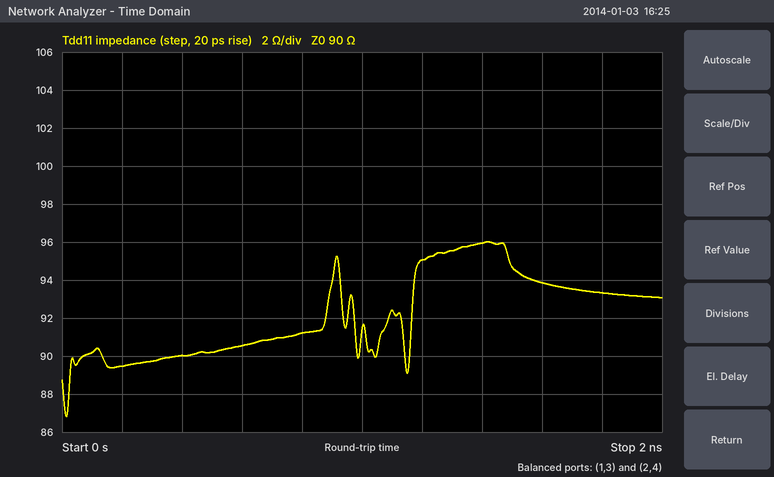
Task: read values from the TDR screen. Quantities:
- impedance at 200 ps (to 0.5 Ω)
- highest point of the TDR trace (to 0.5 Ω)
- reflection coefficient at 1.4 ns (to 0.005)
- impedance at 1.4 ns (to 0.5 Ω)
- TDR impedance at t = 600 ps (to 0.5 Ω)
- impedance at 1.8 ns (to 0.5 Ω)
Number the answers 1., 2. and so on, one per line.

1. 89.5 Ω
2. 96.0 Ω
3. +0.030
4. 96.0 Ω
5. 90.5 Ω
6. 93.5 Ω
